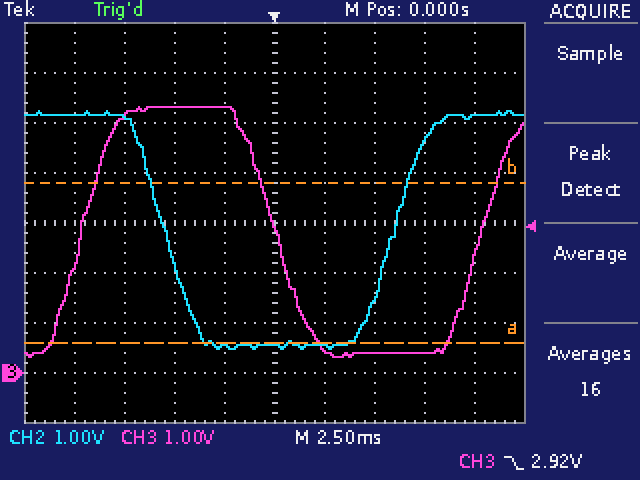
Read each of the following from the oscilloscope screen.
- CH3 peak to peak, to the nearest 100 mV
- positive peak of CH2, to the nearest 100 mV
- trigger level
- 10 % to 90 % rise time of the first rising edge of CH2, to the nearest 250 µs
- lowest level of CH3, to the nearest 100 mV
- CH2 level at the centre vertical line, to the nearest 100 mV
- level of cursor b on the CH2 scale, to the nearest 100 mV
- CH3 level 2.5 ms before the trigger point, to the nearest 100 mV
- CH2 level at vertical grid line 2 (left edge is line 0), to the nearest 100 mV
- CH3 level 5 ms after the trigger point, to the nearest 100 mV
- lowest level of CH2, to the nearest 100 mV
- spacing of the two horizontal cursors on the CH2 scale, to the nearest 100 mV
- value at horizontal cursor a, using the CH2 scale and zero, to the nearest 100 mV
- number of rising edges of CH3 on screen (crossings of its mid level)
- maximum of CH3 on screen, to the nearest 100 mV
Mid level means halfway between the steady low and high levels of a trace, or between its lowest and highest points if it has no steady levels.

5.0 V
5.2 V
2.92 V
3.00 ms
300 mV
600 mV
3.8 V
5.3 V
5.1 V
400 mV
500 mV
3.2 V
600 mV
2
5.3 V
